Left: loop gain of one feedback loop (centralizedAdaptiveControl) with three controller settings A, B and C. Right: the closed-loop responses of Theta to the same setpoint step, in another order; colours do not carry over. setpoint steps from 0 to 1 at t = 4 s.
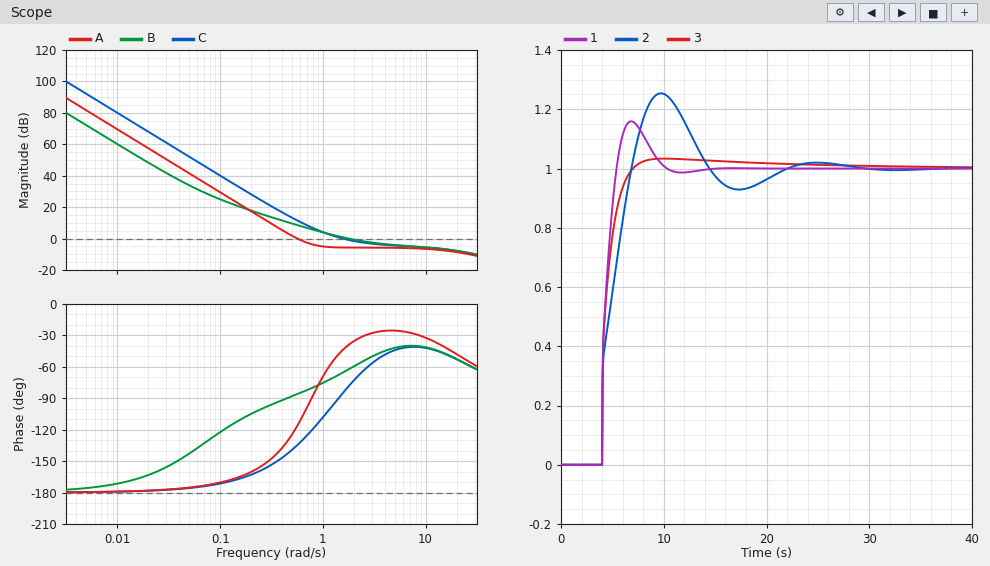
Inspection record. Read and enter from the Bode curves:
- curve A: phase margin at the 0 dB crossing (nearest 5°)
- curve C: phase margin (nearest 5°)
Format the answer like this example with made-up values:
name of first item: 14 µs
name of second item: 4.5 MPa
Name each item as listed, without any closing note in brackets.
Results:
curve A: phase margin at the 0 dB crossing: 65°
curve C: phase margin: 95°
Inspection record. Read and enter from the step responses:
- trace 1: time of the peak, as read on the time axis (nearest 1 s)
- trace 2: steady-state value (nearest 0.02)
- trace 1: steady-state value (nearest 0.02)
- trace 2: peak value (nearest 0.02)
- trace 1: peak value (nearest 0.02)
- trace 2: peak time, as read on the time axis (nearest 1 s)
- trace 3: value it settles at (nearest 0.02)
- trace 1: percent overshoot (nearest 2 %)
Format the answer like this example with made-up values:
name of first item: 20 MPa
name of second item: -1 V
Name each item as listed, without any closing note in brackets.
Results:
trace 1: time of the peak, as read on the time axis: 7 s
trace 2: steady-state value: 1.00
trace 1: steady-state value: 1.00
trace 2: peak value: 1.26
trace 1: peak value: 1.16
trace 2: peak time, as read on the time axis: 10 s
trace 3: value it settles at: 1.00
trace 1: percent overshoot: 16 %
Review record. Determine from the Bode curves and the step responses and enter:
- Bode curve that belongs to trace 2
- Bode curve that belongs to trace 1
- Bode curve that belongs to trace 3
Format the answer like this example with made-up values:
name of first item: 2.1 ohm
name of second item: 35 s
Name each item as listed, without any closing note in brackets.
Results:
Bode curve that belongs to trace 2: A
Bode curve that belongs to trace 1: C
Bode curve that belongs to trace 3: B
